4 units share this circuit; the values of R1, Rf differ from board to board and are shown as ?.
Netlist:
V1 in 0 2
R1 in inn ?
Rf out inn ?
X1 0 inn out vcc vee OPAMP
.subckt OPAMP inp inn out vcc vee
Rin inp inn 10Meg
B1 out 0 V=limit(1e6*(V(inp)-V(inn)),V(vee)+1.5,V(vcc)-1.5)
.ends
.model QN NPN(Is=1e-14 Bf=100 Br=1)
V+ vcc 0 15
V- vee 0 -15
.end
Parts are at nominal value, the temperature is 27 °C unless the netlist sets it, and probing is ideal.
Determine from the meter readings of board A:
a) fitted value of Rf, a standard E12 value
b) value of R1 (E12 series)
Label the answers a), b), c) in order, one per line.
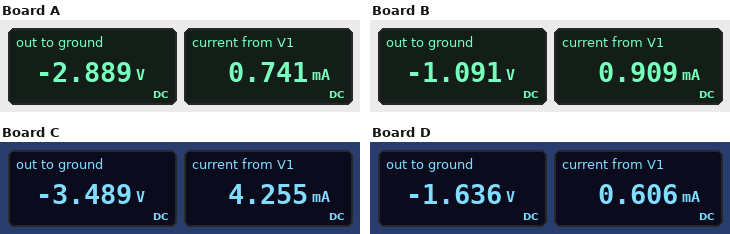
a) 3.9 kΩ
b) 2.7 kΩ
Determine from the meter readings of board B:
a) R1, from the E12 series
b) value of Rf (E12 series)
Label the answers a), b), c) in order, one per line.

a) 2.2 kΩ
b) 1.2 kΩ
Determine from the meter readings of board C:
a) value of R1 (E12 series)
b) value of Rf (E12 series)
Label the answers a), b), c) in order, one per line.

a) 470 Ω
b) 820 Ω
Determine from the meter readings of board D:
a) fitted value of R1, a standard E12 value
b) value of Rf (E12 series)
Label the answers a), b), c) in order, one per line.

a) 3.3 kΩ
b) 2.7 kΩ
